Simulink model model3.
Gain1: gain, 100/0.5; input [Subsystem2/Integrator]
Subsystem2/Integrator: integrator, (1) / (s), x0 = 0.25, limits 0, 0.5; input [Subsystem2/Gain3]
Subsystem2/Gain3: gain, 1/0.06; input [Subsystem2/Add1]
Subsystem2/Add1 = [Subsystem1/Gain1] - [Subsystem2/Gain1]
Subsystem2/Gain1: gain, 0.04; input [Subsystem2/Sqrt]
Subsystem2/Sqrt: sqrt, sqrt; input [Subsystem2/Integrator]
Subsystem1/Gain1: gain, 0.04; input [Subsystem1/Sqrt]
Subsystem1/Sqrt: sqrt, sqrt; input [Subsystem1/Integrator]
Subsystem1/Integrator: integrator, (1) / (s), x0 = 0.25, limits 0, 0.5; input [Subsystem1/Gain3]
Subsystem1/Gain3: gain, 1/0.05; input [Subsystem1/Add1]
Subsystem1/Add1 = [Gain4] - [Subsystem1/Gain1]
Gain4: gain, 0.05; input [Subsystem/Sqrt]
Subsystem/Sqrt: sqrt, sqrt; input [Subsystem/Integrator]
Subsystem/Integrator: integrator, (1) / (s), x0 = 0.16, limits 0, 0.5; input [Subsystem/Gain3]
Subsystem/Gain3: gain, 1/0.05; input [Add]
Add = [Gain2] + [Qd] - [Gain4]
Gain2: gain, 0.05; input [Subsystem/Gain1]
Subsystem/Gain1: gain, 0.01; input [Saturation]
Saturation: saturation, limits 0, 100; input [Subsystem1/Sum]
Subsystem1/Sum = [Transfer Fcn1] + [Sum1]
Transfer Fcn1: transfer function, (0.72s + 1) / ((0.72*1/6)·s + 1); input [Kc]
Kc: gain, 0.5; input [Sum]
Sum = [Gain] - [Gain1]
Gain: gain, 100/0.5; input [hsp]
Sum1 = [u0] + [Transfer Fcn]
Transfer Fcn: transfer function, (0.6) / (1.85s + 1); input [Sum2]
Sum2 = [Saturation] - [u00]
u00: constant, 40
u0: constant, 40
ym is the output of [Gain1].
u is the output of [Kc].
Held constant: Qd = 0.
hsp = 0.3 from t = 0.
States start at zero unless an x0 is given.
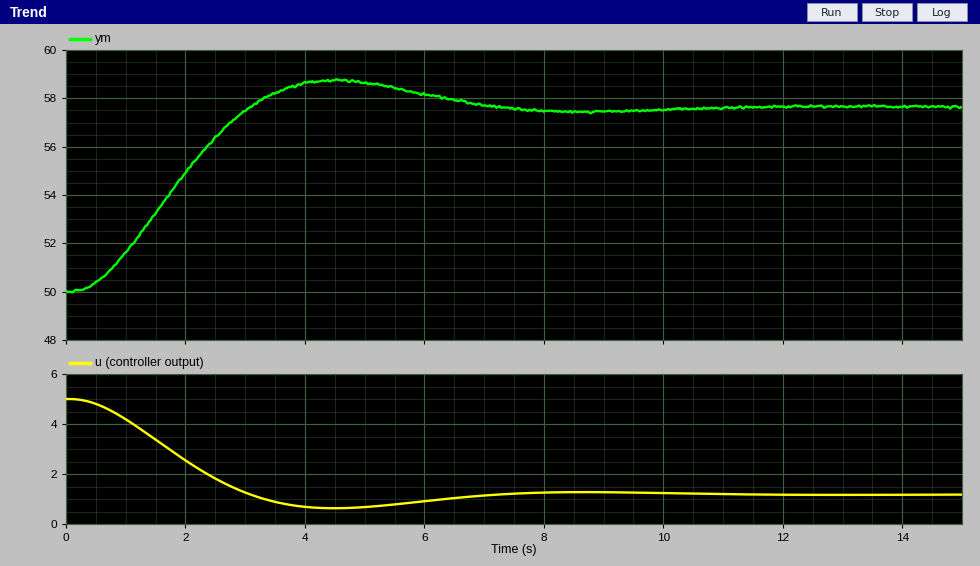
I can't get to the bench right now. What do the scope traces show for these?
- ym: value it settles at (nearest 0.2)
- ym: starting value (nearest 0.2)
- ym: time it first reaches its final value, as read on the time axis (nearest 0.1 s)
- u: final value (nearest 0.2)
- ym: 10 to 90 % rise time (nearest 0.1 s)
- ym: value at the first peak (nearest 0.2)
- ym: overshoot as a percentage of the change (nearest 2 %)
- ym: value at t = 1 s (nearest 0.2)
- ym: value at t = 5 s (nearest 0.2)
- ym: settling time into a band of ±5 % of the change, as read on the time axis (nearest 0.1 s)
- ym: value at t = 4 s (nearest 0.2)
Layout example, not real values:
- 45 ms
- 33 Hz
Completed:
- 57.6
- 50.0
- 3.1 s
- 1.2
- 2.0 s
- 58.8
- 14 %
- 51.6
- 58.6
- 6.3 s
- 58.6
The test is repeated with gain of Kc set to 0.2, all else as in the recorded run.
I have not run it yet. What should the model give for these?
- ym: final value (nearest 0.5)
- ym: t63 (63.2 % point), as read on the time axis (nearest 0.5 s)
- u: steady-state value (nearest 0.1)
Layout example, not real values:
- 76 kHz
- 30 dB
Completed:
- 55.5
- 3.0 s
- 0.9
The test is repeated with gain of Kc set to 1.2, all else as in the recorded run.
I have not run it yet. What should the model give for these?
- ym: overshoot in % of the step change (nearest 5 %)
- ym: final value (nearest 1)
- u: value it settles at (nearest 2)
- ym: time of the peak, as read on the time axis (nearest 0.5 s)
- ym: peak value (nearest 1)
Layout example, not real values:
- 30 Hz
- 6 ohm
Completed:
- 35 %
- 59
- 2
- 3.0 s
- 62
